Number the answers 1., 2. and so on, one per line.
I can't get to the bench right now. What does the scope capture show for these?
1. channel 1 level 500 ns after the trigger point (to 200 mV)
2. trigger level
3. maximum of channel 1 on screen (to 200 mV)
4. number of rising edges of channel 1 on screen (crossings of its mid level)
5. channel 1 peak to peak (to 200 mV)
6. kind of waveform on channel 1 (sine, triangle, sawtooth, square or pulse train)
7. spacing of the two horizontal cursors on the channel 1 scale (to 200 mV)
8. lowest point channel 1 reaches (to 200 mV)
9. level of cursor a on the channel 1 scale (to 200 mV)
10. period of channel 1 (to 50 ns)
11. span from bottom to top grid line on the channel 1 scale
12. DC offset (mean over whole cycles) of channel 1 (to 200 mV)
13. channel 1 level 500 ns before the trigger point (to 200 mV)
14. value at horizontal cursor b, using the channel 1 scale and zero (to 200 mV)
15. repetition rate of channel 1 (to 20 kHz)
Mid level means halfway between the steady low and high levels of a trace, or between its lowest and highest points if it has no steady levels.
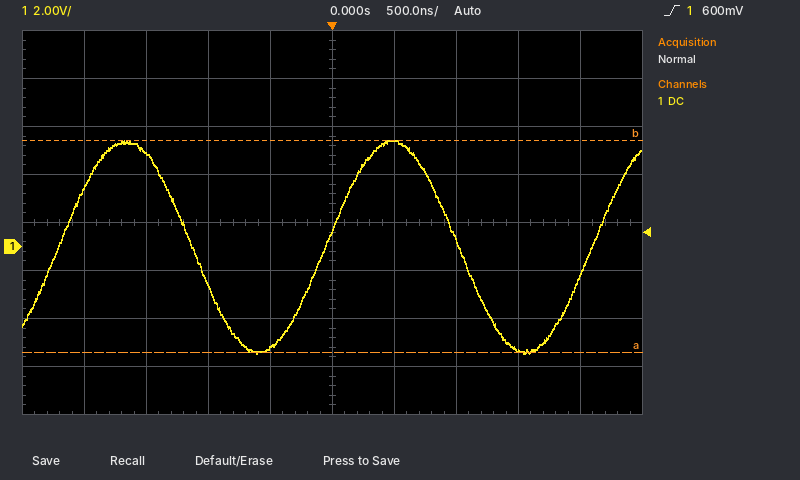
1. 4.4 V
2. 600 mV
3. 4.4 V
4. 3
5. 8.8 V
6. sine
7. 8.8 V
8. -4.4 V
9. -4.4 V
10. 2.15 µs
11. 16 V
12. 0.0 V
13. -4.2 V
14. 4.4 V
15. 460 kHz
